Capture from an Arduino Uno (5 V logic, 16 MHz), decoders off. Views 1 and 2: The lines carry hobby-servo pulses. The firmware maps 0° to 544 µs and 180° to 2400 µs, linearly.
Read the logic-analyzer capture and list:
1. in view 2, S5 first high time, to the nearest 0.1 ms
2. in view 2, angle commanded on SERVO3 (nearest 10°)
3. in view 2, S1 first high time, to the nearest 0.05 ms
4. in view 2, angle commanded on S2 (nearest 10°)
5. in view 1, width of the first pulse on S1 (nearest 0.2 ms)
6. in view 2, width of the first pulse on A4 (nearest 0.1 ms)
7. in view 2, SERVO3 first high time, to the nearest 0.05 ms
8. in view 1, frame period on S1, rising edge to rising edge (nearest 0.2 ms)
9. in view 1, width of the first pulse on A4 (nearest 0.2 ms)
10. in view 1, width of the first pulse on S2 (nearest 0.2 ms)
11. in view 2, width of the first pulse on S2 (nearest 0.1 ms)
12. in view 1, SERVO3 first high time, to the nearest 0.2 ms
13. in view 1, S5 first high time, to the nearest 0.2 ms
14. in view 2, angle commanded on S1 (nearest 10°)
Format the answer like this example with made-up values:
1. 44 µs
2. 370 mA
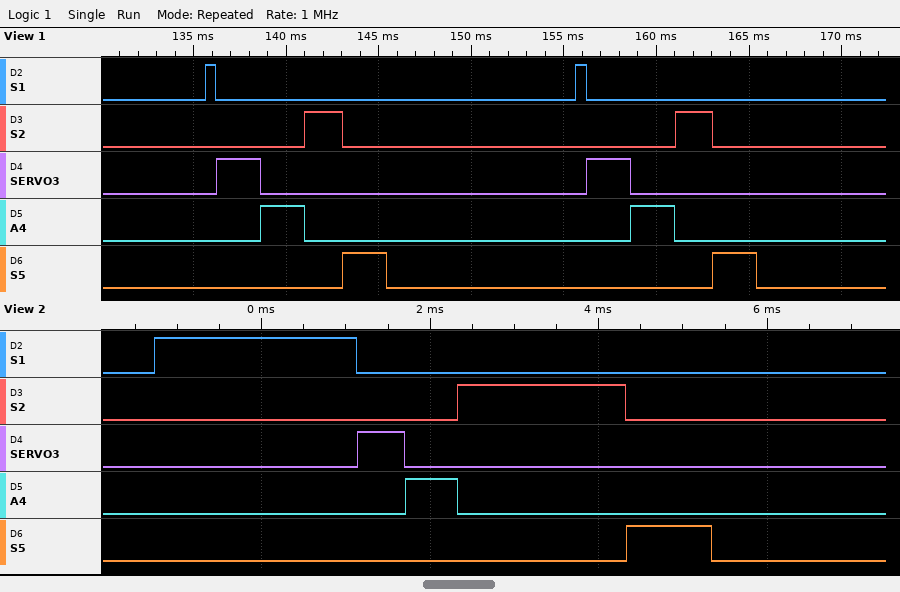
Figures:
1. 1.0 ms
2. 0°
3. 2.40 ms
4. 140°
5. 0.6 ms
6. 0.6 ms
7. 0.55 ms
8. 20.0 ms
9. 2.4 ms
10. 2.0 ms
11. 2.0 ms
12. 2.4 ms
13. 2.4 ms
14. 180°
